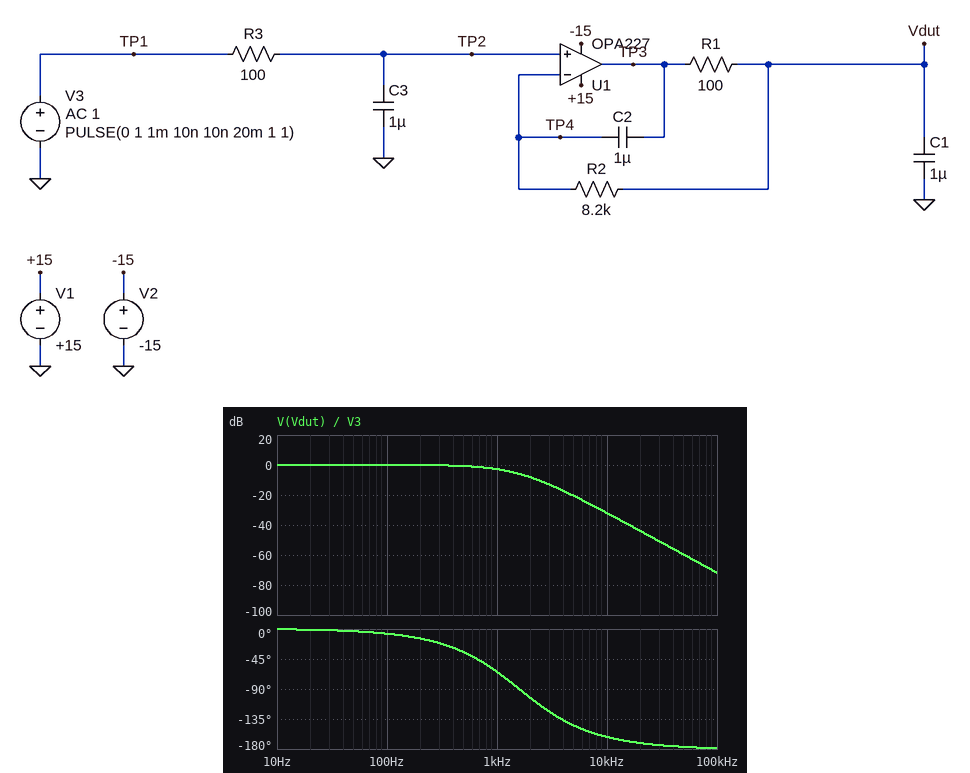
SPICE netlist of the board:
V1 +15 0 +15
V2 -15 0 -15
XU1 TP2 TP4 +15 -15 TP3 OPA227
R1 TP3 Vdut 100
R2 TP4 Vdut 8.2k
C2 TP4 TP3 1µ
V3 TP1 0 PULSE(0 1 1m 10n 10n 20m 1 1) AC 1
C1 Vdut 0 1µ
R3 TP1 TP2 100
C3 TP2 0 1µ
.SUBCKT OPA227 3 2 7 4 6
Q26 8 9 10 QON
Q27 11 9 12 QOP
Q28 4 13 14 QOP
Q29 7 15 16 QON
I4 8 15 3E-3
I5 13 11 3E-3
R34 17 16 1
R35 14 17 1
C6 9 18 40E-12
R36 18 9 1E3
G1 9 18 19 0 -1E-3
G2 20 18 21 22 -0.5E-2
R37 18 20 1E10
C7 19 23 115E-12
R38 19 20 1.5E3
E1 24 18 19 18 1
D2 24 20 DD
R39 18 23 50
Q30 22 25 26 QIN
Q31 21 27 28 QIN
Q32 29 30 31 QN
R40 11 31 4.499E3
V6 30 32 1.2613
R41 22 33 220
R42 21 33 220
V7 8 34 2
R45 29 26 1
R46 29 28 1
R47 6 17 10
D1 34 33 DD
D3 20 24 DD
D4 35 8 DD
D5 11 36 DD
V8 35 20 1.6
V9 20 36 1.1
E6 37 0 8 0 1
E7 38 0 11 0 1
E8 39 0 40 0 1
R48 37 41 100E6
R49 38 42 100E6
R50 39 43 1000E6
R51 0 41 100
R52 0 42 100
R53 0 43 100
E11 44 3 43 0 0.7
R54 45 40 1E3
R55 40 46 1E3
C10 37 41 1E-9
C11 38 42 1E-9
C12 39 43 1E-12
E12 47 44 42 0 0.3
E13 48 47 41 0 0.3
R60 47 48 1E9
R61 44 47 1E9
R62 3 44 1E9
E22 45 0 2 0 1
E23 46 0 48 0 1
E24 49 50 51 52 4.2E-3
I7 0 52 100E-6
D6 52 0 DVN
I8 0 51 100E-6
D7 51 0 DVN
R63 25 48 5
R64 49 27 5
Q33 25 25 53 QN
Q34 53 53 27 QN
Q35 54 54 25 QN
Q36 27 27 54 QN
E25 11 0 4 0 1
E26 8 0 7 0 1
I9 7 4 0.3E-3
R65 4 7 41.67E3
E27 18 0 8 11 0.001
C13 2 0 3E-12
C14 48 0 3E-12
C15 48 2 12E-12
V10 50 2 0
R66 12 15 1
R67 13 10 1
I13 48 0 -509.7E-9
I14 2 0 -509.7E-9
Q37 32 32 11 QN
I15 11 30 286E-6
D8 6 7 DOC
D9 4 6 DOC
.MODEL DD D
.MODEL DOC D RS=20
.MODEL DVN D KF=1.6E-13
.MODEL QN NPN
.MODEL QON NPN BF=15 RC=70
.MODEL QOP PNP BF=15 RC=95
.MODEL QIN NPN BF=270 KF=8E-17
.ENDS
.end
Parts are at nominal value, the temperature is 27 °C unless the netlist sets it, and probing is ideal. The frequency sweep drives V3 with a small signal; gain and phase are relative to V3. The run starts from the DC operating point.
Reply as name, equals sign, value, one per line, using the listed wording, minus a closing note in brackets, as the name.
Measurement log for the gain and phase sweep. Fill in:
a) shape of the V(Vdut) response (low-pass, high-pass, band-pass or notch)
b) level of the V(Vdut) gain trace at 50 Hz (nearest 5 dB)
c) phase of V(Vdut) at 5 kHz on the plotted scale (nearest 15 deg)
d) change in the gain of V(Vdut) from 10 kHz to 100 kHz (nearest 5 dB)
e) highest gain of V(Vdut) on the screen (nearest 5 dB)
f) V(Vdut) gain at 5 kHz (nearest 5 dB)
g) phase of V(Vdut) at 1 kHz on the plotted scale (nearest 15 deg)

shape of the V(Vdut) response = low-pass
level of the V(Vdut) gain trace at 50 Hz = 0 dB
phase of V(Vdut) at 5 kHz on the plotted scale = -150 deg
change in the gain of V(Vdut) from 10 kHz to 100 kHz = -40 dB
highest gain of V(Vdut) on the screen = 0 dB
V(Vdut) gain at 5 kHz = -20 dB
phase of V(Vdut) at 1 kHz on the plotted scale = -60 deg
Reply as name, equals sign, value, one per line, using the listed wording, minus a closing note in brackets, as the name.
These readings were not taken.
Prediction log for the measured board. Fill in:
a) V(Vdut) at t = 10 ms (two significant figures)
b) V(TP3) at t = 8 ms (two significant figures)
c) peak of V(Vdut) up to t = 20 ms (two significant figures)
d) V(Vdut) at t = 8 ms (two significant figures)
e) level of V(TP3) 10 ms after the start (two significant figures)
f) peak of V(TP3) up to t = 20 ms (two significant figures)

V(Vdut) at t = 10 ms = 1.0 V
V(TP3) at t = 8 ms = 1.0 V
peak of V(Vdut) up to t = 20 ms = 1.0 V
V(Vdut) at t = 8 ms = 1.0 V
level of V(TP3) 10 ms after the start = 1.0 V
peak of V(TP3) up to t = 20 ms = 1.0 V
